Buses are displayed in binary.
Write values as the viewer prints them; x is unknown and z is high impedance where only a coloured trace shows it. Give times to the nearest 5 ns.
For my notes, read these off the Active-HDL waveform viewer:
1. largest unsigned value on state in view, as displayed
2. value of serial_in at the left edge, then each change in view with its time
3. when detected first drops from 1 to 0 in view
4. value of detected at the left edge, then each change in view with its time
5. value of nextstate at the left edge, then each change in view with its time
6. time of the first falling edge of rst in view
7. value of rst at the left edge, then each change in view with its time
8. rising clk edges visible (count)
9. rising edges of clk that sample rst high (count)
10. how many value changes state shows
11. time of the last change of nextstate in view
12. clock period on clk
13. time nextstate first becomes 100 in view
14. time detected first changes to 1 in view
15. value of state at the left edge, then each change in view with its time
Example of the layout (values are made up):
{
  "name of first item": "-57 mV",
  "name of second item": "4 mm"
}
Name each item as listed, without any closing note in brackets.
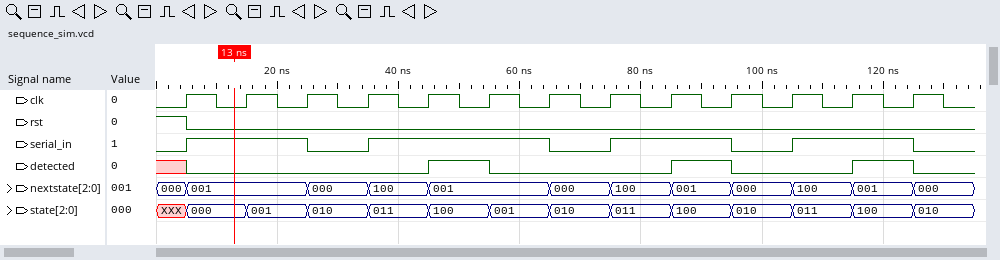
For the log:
{
  "largest unsigned value on state in view, as displayed": "100",
  "value of serial_in at the left edge, then each change in view with its time": "0, 1 at 5 ns, 0 at 25 ns, 1 at 35 ns, 0 at 65 ns, 1 at 75 ns, 0 at 95 ns, 1 at 105 ns, 0 at 125 ns",
  "when detected first drops from 1 to 0 in view": "55 ns",
  "value of detected at the left edge, then each change in view with its time": "x, 0 at 5 ns, 1 at 45 ns, 0 at 55 ns, 1 at 85 ns, 0 at 95 ns, 1 at 115 ns, 0 at 125 ns",
  "value of nextstate at the left edge, then each change in view with its time": "000, 001 at 5 ns, 000 at 25 ns, 100 at 35 ns, 001 at 45 ns, 000 at 65 ns, 100 at 75 ns, 001 at 85 ns, 000 at 95 ns, 100 at 105 ns, 001 at 115 ns, 000 at 125 ns",
  "time of the first falling edge of rst in view": "5 ns",
  "value of rst at the left edge, then each change in view with its time": "1, 0 at 5 ns",
  "rising clk edges visible": "13",
  "rising edges of clk that sample rst high": "1",
  "how many value changes state shows": "13",
  "time of the last change of nextstate in view": "125 ns",
  "clock period on clk": "10 ns",
  "time nextstate first becomes 100 in view": "35 ns",
  "time detected first changes to 1 in view": "45 ns",
  "value of state at the left edge, then each change in view with its time": "XXX, 000 at 5 ns, 001 at 15 ns, 010 at 25 ns, 011 at 35 ns, 100 at 45 ns, 001 at 55 ns, 010 at 65 ns, 011 at 75 ns, 100 at 85 ns, 010 at 95 ns, 011 at 105 ns, 100 at 115 ns, 010 at 125 ns"
}
